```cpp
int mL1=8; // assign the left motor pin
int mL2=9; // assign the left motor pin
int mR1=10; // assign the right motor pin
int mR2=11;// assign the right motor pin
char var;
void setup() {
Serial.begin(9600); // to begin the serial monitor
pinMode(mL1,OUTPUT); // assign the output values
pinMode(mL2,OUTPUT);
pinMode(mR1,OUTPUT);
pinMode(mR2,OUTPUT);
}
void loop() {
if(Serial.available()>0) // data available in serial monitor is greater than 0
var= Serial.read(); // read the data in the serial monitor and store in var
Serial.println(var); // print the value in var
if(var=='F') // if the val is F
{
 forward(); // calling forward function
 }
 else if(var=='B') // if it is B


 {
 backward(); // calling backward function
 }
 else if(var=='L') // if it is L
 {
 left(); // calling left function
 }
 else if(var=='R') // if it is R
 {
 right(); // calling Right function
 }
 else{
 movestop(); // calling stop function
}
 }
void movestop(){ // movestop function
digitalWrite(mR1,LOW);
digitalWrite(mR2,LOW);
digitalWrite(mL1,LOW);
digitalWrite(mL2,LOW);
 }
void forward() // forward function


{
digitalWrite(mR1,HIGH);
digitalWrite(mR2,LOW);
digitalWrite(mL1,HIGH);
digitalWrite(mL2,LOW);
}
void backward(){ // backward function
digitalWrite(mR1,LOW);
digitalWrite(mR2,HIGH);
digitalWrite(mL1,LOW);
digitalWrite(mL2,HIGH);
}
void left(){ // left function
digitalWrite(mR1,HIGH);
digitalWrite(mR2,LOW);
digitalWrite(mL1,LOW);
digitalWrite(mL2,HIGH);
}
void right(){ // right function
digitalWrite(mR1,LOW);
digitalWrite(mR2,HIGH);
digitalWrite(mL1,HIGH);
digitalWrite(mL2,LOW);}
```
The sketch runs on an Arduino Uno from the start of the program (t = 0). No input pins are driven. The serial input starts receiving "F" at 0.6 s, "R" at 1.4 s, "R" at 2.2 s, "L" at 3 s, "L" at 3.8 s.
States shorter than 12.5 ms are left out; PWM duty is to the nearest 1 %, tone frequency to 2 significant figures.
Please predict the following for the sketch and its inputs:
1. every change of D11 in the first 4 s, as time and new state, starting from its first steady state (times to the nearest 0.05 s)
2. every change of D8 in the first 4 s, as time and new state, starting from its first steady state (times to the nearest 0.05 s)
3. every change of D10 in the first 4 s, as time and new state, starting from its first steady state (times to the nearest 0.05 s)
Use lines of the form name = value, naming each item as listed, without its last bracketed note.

every change of D11 in the first 4 s, as time and new state, starting from its first steady state = 0 s low; 1.4 s high; 3 s low
every change of D8 in the first 4 s, as time and new state, starting from its first steady state = 0 s low; 0.6 s high; 3 s low
every change of D10 in the first 4 s, as time and new state, starting from its first steady state = 0 s low; 0.6 s high; 1.4 s low; 3 s high
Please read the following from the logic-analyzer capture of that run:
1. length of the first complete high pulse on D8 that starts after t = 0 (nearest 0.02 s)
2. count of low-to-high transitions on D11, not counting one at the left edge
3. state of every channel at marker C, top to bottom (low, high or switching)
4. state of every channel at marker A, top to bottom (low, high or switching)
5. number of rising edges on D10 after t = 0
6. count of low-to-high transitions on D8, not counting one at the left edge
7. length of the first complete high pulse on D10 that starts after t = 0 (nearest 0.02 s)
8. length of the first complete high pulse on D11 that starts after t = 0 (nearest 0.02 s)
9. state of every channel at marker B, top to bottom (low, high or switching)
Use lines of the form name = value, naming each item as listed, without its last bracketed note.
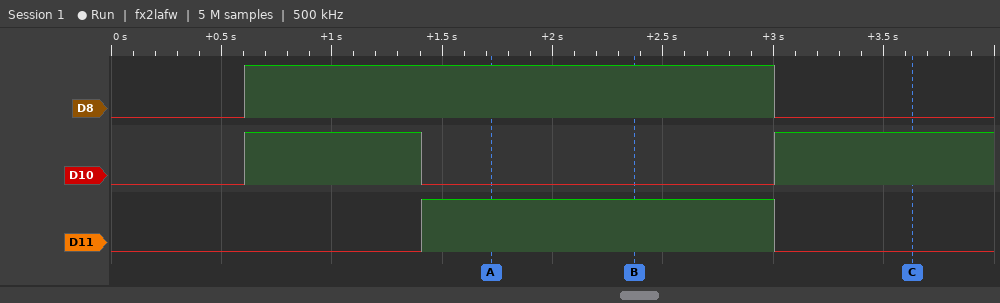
length of the first complete high pulse on D8 that starts after t = 0 = 2.40 s
count of low-to-high transitions on D11, not counting one at the left edge = 1
state of every channel at marker C, top to bottom = D8 low, D10 high, D11 low
state of every channel at marker A, top to bottom = D8 high, D10 low, D11 high
number of rising edges on D10 after t = 0 = 2
count of low-to-high transitions on D8, not counting one at the left edge = 1
length of the first complete high pulse on D10 that starts after t = 0 = 0.80 s
length of the first complete high pulse on D11 that starts after t = 0 = 1.60 s
state of every channel at marker B, top to bottom = D8 high, D10 low, D11 high
